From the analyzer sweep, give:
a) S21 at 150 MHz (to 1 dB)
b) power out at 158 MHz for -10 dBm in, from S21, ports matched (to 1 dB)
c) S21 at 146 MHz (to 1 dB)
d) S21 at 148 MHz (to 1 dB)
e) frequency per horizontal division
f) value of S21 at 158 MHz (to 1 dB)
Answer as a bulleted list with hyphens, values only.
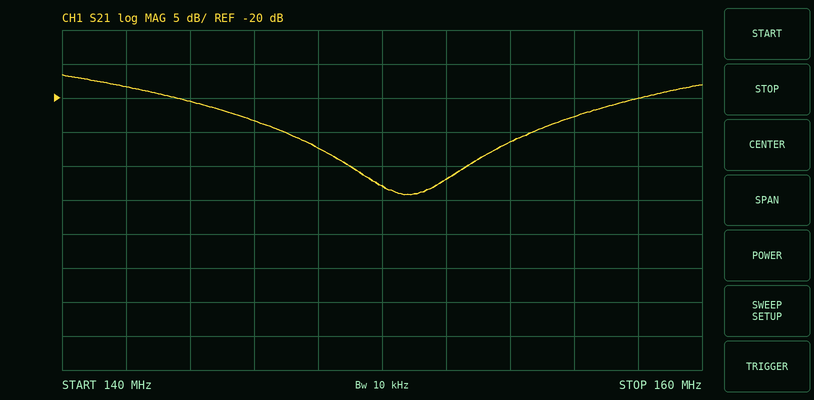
- -33 dB
- -30 dBm
- -23 dB
- -27 dB
- 2 MHz
- -20 dB
